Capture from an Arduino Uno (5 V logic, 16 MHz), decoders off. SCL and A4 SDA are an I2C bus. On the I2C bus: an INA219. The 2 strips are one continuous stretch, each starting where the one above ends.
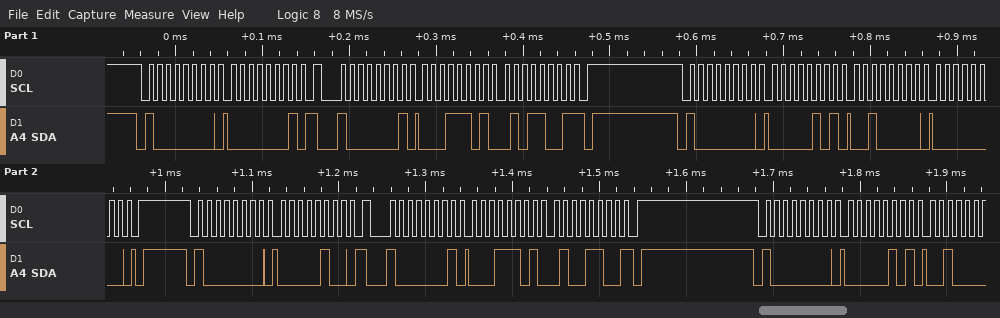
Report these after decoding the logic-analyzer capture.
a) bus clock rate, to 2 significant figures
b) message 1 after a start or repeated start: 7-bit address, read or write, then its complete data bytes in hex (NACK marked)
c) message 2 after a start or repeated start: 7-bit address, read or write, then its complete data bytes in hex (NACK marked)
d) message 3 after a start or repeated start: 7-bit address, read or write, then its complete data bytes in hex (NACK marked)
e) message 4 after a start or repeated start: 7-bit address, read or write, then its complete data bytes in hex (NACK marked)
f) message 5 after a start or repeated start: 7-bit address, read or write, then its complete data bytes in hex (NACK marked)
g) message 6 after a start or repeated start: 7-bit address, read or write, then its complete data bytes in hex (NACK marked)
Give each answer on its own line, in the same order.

100 kHz
0x40 write: 01
0x40 read: 1D 59 NACK
0x40 write: 05 20 00
0x40 write: 04
0x40 read: 1D 4C NACK
0x40 write: 05
